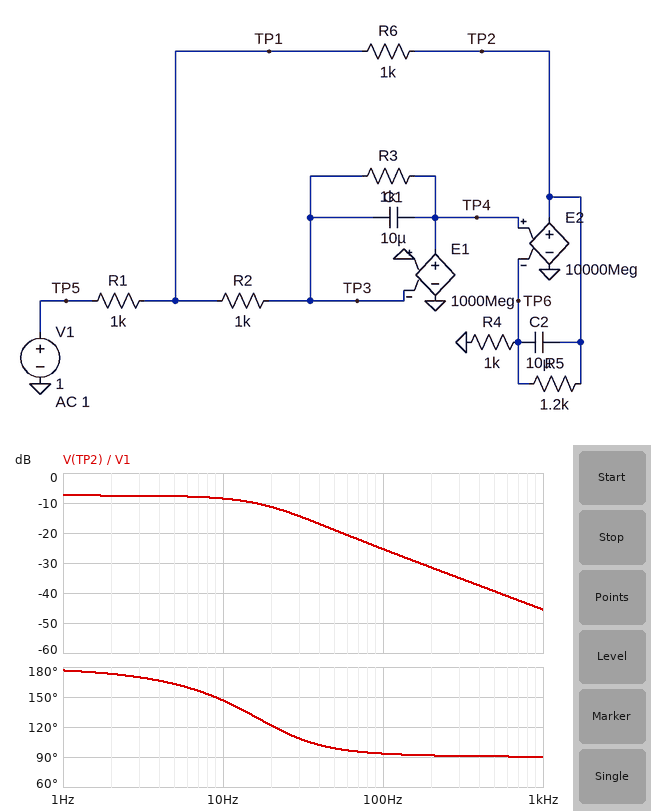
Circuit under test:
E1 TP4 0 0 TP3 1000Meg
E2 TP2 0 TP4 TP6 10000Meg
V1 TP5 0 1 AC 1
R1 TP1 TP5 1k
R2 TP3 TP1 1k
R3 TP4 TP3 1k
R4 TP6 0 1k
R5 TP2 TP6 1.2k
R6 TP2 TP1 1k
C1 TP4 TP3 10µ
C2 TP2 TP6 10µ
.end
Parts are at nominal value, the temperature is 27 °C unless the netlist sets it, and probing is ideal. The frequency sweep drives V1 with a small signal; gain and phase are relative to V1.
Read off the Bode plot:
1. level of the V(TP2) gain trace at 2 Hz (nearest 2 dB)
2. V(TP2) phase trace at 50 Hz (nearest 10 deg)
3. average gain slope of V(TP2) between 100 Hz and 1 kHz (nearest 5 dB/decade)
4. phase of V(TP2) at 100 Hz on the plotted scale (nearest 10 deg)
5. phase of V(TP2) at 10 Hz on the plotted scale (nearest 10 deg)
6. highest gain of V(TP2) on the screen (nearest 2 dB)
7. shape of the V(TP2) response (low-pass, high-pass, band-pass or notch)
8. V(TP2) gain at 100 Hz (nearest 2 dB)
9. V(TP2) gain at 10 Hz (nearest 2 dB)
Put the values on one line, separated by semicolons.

-8 dB; 100 deg; -20 dB/decade; 90 deg; 150 deg; -8 dB; low-pass; -26 dB; -8 dB
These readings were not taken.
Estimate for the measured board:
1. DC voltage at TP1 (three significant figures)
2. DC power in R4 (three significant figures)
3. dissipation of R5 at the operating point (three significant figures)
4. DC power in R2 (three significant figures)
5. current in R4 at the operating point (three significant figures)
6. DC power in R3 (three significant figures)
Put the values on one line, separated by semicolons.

192 mV; 37.0 µW; 44.4 µW; 37.0 µW; 192 µA; 37.0 µW
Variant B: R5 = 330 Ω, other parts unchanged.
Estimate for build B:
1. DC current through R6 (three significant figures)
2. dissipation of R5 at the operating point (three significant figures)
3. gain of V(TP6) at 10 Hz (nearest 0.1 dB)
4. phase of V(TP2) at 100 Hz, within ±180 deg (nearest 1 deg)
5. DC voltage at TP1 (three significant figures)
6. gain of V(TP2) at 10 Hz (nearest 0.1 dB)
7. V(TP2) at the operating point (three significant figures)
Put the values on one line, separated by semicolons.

538 µA; 17.6 µW; -13.4 dB; 95 deg; 231 mV; -11.0 dB; -307 mV
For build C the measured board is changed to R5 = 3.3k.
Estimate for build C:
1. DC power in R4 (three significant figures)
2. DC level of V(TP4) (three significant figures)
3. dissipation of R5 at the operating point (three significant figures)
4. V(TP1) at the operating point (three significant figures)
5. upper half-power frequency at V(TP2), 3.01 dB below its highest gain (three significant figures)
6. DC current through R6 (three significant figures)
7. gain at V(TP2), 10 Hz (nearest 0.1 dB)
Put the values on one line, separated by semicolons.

18.8 µW; -137 mV; 61.9 µW; 137 mV; 11.3 Hz; 726 µA; -7.0 dB
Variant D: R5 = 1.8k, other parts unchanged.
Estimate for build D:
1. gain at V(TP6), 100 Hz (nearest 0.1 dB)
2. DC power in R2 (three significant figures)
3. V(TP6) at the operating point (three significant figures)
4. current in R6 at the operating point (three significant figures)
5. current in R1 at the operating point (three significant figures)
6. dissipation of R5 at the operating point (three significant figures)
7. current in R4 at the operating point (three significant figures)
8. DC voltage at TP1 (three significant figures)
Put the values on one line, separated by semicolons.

-25.6 dB; 29.7 µW; -172 mV; 655 µA; 828 µA; 53.5 µW; 172 µA; 172 mV
